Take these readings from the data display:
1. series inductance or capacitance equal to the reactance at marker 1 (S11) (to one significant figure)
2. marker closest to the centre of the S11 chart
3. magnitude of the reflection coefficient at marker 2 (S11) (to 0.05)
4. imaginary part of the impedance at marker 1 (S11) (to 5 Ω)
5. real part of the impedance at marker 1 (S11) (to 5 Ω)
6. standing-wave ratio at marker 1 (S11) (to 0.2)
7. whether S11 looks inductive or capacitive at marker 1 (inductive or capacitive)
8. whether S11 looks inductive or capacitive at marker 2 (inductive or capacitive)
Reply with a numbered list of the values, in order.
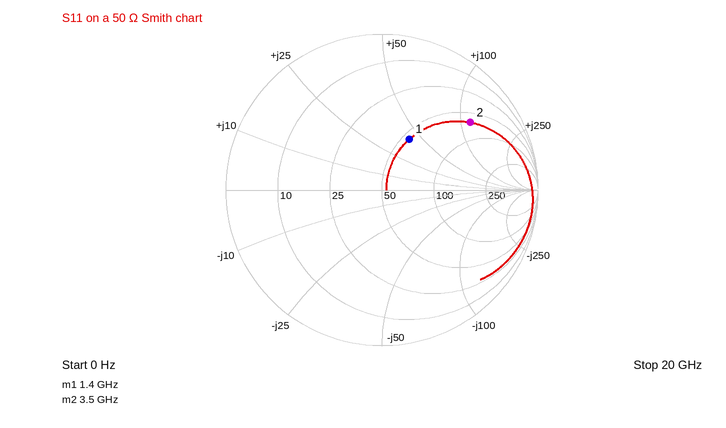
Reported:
1. 5 nH
2. marker 1
3. 0.70
4. +40 Ω
5. 55 Ω
6. 2.2
7. inductive
8. inductive
